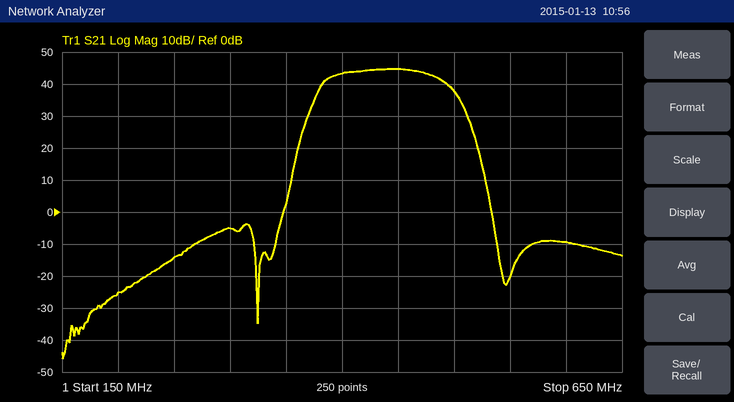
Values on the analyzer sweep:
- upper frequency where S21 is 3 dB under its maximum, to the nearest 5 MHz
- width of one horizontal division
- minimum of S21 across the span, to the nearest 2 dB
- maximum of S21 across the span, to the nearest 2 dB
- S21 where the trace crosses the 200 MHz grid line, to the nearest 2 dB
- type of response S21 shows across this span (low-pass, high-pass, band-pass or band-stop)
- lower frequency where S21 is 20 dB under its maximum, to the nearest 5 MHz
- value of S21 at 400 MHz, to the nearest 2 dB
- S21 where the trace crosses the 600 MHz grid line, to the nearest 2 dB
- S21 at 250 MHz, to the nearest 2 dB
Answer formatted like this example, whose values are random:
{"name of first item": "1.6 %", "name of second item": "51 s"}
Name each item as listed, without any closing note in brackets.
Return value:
{"upper frequency where S21 is 3 dB under its maximum, to the nearest 5 MHz": "485 MHz", "width of one horizontal division": "50 MHz", "minimum of S21 across the span, to the nearest 2 dB": "-46 dB", "maximum of S21 across the span, to the nearest 2 dB": "44 dB", "S21 where the trace crosses the 200 MHz grid line, to the nearest 2 dB": "-26 dB", "type of response S21 shows across this span": "band-pass", "lower frequency where S21 is 20 dB under its maximum, to the nearest 5 MHz": "365 MHz", "value of S21 at 400 MHz, to the nearest 2 dB": "44 dB", "S21 where the trace crosses the 600 MHz grid line, to the nearest 2 dB": "-10 dB", "S21 at 250 MHz, to the nearest 2 dB": "-14 dB"}
